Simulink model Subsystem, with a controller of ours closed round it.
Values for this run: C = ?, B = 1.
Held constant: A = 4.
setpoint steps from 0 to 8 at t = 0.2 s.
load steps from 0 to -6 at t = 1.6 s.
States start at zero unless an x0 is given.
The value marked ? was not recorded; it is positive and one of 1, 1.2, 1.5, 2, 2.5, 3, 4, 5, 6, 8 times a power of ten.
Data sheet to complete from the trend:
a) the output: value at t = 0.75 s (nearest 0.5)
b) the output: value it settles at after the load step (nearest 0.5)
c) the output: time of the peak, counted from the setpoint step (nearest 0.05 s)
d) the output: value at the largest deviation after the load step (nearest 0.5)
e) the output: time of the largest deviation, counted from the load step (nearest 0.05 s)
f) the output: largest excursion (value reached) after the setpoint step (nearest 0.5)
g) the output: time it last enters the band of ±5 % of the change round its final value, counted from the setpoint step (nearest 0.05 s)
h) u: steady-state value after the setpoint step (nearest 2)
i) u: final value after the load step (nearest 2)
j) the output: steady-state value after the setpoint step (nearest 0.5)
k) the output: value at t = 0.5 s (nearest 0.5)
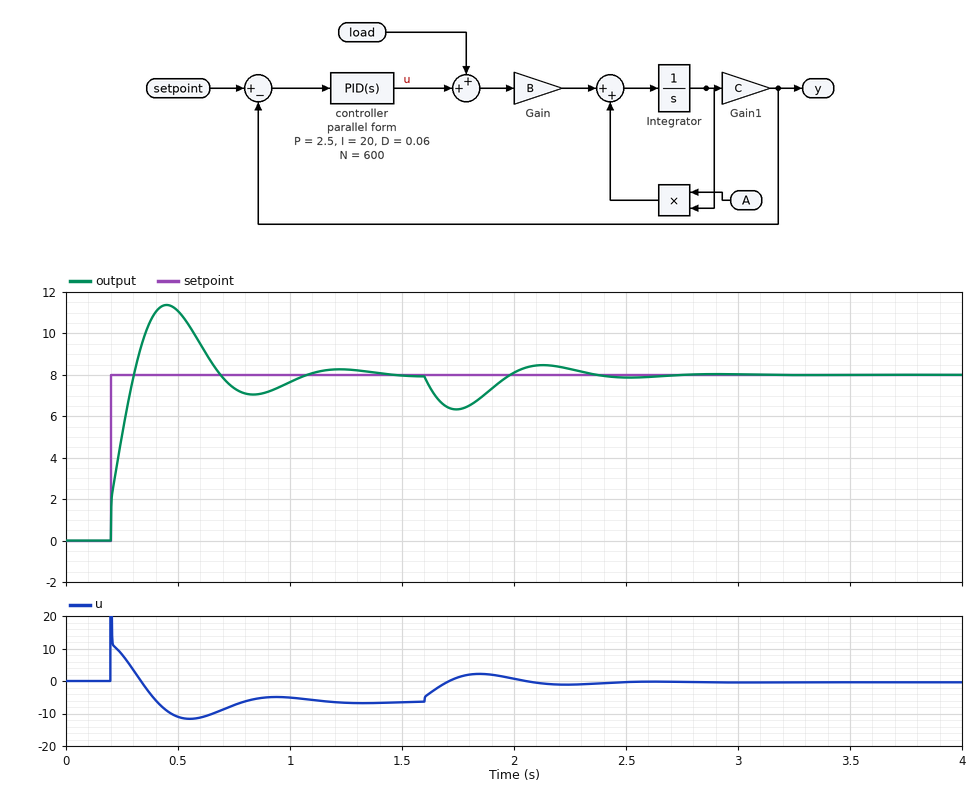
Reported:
7.5
8.0
0.25 s
6.5
0.15 s
11.5
0.80 s
-6
0
8.0
11.0
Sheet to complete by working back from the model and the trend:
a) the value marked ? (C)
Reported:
5
